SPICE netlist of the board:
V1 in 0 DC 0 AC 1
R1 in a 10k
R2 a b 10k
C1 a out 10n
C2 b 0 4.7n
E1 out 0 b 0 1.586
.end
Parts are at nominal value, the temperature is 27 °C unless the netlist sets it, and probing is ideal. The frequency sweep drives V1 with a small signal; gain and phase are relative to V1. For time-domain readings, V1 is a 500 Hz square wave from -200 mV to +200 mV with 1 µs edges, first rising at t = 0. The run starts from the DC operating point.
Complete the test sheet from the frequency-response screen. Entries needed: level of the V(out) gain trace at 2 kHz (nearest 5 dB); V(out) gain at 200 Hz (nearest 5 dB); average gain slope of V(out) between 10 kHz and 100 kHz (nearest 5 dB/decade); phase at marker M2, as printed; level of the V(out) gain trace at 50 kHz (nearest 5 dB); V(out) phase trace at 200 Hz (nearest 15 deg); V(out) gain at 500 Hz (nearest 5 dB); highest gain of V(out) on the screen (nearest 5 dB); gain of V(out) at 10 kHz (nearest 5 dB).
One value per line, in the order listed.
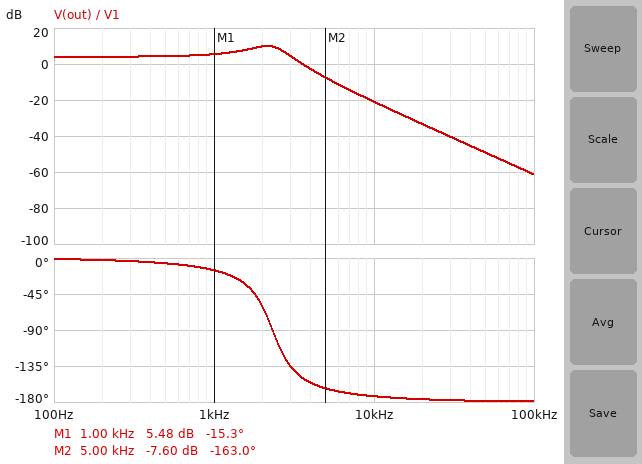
10 dB
5 dB
-40 dB/decade
-163.0 deg
-50 dB
0 deg
5 dB
10 dB
-20 dB
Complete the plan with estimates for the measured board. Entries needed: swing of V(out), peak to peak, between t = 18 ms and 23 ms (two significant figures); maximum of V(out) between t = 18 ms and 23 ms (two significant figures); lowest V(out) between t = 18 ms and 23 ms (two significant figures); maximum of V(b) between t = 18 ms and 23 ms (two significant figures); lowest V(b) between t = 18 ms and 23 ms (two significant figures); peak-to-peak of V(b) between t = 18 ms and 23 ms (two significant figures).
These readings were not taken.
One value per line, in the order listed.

1.2 V
590 mV
-590 mV
370 mV
-370 mV
740 mV
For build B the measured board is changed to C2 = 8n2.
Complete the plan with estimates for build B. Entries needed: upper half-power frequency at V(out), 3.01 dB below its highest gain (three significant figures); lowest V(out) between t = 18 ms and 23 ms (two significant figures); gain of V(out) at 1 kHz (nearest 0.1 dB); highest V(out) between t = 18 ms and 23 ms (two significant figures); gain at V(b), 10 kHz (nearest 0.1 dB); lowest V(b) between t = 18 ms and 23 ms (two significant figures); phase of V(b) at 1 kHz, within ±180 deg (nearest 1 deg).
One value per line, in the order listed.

1.98 kHz
-380 mV
4.5 dB
380 mV
-30.1 dB
-240 mV
-44 deg
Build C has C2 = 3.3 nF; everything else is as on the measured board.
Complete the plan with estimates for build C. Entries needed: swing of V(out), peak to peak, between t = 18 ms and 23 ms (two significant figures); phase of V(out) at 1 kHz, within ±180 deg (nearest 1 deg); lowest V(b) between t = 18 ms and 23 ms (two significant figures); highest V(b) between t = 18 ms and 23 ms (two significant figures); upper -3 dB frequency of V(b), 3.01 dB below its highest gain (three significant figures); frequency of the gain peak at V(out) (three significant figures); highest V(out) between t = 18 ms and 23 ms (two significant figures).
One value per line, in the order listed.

1.6 V
-3 deg
-510 mV
510 mV
2.93 kHz
2.76 kHz
810 mV
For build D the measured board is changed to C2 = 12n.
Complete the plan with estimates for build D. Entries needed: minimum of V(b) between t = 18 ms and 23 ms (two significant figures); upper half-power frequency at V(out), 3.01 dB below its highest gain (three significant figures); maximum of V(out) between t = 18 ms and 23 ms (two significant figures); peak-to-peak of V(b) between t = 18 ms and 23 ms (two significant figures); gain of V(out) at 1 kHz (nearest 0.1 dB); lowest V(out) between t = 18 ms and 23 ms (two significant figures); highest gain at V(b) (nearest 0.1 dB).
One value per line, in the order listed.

-200 mV
1.21 kHz
320 mV
410 mV
2.0 dB
-320 mV
0 dB
